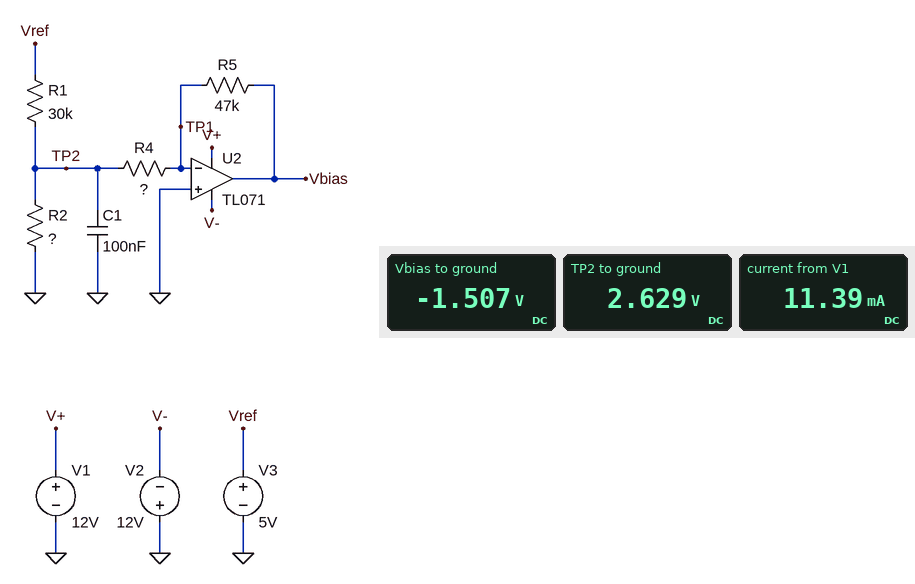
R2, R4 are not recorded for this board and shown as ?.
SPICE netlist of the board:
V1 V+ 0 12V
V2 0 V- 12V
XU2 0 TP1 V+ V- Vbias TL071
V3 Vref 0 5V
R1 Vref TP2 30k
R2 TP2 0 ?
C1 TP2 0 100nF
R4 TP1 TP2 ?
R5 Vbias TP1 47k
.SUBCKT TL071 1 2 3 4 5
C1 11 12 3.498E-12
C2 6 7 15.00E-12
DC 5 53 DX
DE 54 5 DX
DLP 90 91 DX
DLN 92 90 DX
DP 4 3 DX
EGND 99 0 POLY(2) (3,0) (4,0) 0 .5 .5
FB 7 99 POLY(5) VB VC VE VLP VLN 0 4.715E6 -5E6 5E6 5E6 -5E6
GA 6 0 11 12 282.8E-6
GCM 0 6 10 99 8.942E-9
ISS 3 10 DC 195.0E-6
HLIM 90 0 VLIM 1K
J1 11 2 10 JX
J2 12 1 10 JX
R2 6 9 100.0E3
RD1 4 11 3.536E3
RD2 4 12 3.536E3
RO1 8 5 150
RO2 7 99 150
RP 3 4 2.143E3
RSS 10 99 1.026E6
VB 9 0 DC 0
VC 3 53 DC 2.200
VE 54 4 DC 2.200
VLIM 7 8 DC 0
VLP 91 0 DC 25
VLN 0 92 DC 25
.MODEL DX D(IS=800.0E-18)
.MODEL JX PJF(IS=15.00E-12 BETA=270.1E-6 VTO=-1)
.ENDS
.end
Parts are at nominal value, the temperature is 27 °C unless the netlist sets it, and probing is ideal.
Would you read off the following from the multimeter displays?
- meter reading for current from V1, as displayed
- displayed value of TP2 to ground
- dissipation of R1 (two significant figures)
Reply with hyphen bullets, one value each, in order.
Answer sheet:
- 11.39 mA
- 2.629 V
- 190 µW
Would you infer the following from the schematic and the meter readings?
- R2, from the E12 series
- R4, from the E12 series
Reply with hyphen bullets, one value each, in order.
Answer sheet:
- 56 kΩ
- 82 kΩ
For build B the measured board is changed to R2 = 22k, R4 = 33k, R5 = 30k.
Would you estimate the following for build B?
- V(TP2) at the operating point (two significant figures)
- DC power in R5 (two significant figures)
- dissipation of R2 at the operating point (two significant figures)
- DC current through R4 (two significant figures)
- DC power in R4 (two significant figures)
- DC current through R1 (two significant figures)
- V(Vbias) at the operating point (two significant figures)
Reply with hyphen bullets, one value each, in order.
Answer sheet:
- 1.5 V
- 64 µW
- 110 µW
- 46 µA
- 71 µW
- 120 µA
- -1.4 V
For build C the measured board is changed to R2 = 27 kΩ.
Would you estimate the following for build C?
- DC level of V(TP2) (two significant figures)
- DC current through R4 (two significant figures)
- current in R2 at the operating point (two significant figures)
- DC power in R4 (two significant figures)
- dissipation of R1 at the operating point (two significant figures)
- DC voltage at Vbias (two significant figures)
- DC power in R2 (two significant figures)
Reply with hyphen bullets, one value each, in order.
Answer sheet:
- 2.0 V
- 25 µA
- 75 µA
- 50 µW
- 300 µW
- -1.2 V
- 150 µW
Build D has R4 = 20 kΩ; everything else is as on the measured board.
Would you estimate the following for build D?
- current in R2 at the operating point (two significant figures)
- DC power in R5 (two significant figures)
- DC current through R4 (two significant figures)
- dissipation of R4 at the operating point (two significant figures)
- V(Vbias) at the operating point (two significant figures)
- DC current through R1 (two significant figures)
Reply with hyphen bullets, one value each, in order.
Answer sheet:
- 29 µA
- 320 µW
- 82 µA
- 140 µW
- -3.9 V
- 110 µA
